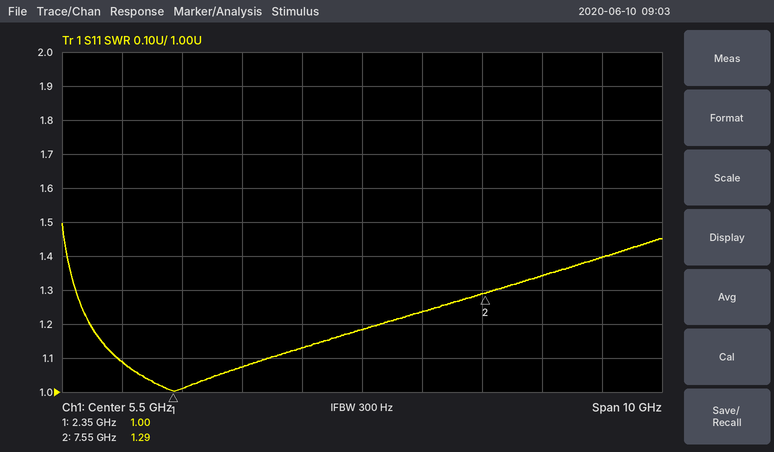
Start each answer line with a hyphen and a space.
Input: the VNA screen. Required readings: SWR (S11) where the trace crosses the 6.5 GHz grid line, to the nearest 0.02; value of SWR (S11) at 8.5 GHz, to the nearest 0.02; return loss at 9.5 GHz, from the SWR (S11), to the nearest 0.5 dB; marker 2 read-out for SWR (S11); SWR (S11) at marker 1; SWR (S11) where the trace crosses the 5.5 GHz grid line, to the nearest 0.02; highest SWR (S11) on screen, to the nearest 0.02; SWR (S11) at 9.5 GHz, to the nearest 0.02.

- 1.24
- 1.34
- 15.5 dB
- 1.29
- 1.00
- 1.18
- 1.50
- 1.40
